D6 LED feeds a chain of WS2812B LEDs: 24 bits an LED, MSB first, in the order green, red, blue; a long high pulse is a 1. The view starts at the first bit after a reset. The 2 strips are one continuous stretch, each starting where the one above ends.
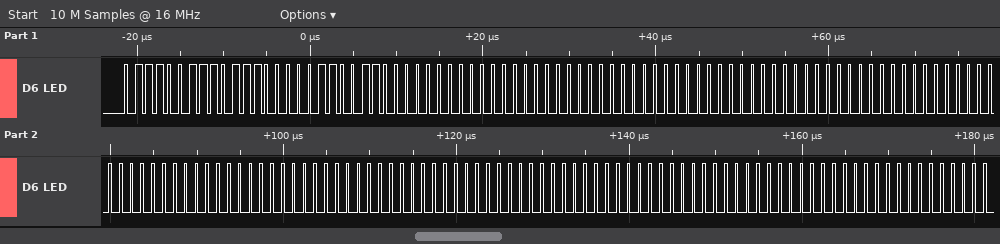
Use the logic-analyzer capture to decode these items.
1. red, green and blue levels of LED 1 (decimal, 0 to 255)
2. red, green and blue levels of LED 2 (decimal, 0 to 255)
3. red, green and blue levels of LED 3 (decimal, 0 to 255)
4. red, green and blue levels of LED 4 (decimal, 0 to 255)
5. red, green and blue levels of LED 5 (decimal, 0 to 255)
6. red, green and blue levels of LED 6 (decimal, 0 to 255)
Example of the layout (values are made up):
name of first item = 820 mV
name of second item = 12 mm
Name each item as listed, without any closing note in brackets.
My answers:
red, green and blue levels of LED 1 = 184, 115, 51
red, green and blue levels of LED 2 = 0, 0, 0
red, green and blue levels of LED 3 = 0, 0, 0
red, green and blue levels of LED 4 = 0, 0, 0
red, green and blue levels of LED 5 = 0, 0, 0
red, green and blue levels of LED 6 = 0, 0, 0
